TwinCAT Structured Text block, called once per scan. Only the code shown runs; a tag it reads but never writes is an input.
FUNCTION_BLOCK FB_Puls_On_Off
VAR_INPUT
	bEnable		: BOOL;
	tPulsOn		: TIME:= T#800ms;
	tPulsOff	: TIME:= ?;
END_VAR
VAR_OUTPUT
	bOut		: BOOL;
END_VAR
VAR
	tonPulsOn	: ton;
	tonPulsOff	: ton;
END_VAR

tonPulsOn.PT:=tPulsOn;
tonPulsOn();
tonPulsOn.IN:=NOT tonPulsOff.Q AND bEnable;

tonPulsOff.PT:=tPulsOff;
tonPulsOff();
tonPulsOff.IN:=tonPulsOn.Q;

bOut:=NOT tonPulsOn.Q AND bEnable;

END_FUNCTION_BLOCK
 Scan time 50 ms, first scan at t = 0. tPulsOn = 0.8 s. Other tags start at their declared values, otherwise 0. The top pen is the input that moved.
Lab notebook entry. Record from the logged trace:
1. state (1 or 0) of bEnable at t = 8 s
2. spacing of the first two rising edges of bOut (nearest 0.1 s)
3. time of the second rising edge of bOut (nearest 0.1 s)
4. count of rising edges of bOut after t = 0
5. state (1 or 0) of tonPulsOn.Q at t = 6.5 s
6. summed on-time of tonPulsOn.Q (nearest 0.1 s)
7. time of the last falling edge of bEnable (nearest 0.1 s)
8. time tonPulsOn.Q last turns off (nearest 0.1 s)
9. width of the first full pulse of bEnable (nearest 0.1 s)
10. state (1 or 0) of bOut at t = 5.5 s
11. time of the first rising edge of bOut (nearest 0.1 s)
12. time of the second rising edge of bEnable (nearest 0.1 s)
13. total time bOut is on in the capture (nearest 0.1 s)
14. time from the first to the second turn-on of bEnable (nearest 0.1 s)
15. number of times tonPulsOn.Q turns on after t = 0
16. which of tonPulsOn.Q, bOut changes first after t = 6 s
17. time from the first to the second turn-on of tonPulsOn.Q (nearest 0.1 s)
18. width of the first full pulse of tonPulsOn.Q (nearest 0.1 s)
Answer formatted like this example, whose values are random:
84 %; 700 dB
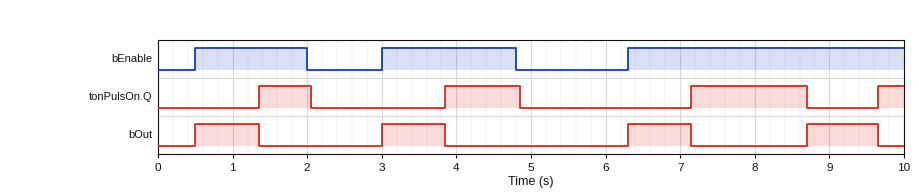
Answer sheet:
1; 2.5 s; 3.0 s; 4; 0; 3.6 s; 4.8 s; 8.7 s; 1.5 s; 0; 0.5 s; 3.0 s; 3.5 s; 2.5 s; 4; bOut; 2.5 s; 0.7 s
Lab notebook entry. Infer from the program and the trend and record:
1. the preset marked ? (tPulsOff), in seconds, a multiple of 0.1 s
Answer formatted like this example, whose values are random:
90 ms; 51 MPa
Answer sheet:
1.4 s
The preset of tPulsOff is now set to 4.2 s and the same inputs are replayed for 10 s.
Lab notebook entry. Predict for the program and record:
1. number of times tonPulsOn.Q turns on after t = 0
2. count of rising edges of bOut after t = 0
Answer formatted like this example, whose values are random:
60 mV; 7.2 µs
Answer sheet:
3; 3
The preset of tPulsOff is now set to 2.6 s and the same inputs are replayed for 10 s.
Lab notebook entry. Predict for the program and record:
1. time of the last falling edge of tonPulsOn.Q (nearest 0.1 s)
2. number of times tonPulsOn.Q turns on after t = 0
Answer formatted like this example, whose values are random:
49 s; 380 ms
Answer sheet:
9.9 s; 3
